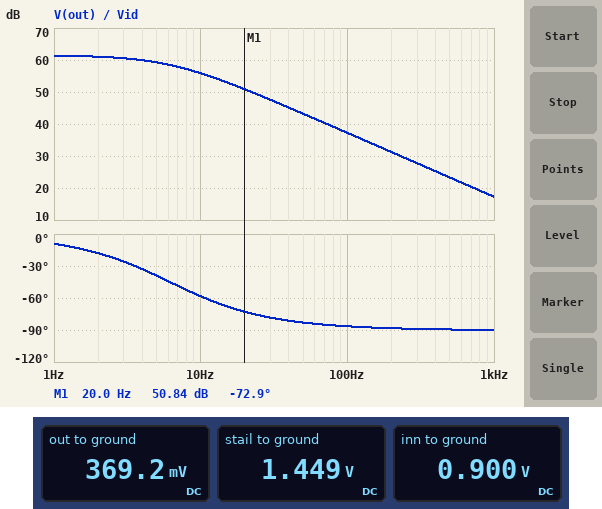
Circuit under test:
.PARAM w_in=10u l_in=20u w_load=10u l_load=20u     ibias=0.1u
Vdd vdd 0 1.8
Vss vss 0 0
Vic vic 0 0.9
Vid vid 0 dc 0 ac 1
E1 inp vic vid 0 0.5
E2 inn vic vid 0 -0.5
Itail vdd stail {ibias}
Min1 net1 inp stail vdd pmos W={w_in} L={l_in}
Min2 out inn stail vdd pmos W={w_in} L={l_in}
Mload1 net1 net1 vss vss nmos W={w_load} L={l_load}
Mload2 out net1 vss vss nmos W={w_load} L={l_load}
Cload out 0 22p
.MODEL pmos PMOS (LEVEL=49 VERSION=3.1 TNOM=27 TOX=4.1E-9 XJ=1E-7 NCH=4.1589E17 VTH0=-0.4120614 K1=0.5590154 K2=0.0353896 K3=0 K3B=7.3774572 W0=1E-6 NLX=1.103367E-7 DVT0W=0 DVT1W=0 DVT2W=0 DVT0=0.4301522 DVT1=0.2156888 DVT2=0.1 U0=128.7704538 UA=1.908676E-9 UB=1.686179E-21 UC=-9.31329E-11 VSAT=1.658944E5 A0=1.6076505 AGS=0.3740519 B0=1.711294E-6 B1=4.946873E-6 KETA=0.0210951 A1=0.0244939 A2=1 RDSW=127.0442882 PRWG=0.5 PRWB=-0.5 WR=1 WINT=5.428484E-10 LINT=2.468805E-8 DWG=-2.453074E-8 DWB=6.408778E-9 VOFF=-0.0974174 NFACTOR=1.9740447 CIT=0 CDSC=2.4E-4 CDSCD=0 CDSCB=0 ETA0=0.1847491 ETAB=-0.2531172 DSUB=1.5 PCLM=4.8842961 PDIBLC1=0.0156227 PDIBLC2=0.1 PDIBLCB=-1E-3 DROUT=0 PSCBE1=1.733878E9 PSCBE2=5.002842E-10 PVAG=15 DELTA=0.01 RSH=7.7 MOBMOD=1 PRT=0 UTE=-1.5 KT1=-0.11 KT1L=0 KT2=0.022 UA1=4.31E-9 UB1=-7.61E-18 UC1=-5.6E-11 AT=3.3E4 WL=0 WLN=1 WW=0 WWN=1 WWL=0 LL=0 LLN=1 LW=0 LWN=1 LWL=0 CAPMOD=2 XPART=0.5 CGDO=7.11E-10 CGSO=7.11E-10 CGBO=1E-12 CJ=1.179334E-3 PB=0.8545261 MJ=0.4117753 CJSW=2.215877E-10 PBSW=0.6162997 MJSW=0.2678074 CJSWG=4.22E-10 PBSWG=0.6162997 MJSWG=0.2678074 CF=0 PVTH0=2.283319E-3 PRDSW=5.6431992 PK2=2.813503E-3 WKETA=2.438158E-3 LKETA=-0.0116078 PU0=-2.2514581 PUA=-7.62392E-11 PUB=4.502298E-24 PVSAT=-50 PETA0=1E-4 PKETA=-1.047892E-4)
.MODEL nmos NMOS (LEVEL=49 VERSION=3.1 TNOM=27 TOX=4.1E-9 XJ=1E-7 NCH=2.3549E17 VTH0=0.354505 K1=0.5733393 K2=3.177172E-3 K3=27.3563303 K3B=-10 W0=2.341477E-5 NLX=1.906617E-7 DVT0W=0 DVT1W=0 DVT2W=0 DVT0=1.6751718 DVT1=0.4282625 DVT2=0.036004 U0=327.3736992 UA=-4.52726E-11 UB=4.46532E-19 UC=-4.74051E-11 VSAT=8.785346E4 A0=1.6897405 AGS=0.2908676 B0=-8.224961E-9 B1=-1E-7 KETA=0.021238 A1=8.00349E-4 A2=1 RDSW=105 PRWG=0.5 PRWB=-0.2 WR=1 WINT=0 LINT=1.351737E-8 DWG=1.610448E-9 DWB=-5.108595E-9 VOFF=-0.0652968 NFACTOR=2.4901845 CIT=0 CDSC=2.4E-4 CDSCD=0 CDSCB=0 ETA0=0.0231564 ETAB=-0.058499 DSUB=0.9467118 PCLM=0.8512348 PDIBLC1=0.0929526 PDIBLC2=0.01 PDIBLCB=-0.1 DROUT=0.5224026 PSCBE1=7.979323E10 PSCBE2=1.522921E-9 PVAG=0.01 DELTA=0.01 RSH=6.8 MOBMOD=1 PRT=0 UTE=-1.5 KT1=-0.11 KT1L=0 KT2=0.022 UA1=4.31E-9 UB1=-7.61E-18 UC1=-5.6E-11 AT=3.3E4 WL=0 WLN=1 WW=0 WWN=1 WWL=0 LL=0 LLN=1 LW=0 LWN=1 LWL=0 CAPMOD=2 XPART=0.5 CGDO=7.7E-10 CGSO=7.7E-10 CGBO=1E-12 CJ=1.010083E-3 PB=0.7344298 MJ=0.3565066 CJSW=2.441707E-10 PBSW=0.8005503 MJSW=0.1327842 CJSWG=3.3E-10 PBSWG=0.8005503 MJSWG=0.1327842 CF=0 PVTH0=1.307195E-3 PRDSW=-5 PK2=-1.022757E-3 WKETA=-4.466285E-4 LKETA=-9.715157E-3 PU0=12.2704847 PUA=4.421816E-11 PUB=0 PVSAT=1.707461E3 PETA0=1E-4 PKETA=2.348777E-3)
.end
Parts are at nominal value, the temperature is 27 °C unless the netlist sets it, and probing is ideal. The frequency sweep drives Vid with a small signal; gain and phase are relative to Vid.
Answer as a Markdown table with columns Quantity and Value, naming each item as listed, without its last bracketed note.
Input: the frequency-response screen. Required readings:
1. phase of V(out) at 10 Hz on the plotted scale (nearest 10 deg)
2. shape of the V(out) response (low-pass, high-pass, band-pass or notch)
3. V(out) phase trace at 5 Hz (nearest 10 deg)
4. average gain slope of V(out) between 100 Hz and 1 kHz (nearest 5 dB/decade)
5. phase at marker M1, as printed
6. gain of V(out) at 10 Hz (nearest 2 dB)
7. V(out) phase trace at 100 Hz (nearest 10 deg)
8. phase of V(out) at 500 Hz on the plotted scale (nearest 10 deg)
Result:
| Quantity | Value |
|---|---|
| phase of V(out) at 10 Hz on the plotted scale | -60 deg |
| shape of the V(out) response | low-pass |
| V(out) phase trace at 5 Hz | -40 deg |
| average gain slope of V(out) between 100 Hz and 1 kHz | -20 dB/decade |
| phase at marker M1, as printed | -72.9 deg |
| gain of V(out) at 10 Hz | 56 dB |
| V(out) phase trace at 100 Hz | -90 deg |
| phase of V(out) at 500 Hz on the plotted scale | -90 deg |
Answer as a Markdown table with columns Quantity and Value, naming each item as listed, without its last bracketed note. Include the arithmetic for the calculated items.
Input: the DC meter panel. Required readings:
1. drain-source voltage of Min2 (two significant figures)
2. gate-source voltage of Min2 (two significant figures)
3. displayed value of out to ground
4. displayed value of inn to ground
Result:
| Quantity | Value |
|---|---|
| drain-source voltage of Min2 | 369.2 mV - 1.449 V = -1.1 V |
| gate-source voltage of Min2 | 900 mV - 1.449 V = -550 mV |
| displayed value of out to ground | 369.2 mV |
| displayed value of inn to ground | 0.900 V |
